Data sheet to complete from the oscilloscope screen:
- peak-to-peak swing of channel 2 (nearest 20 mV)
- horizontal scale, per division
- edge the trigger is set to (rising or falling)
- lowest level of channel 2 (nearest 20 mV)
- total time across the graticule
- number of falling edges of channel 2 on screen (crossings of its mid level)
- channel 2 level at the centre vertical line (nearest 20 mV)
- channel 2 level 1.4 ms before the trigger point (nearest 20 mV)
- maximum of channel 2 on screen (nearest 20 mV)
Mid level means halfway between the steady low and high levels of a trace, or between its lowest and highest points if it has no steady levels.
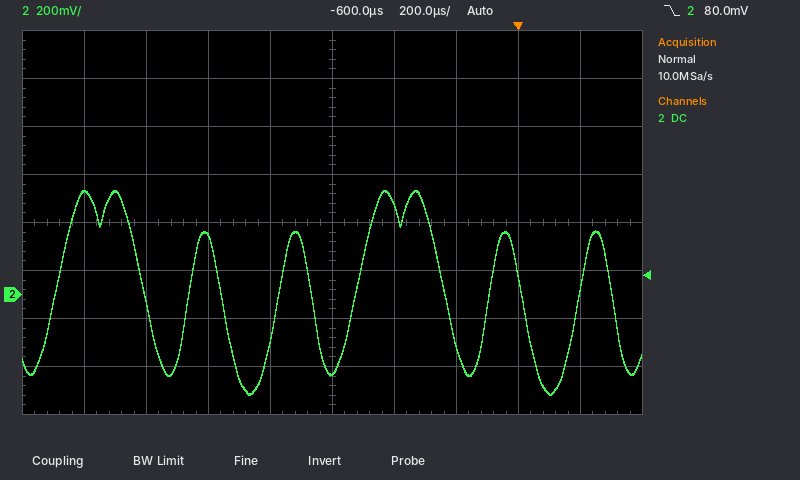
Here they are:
860 mV
200 µs
falling
-420 mV
2 ms
6
-320 mV
420 mV
440 mV
